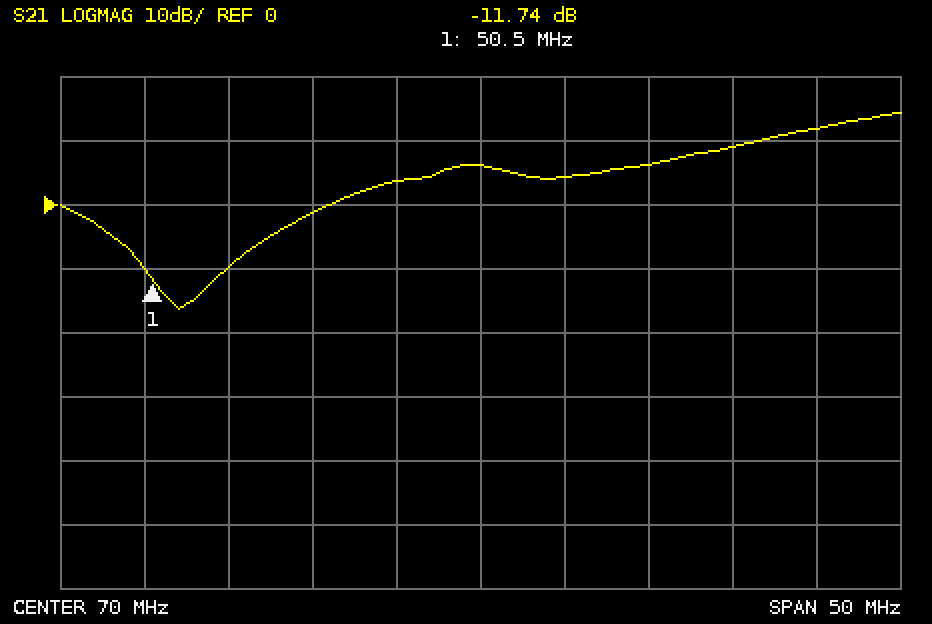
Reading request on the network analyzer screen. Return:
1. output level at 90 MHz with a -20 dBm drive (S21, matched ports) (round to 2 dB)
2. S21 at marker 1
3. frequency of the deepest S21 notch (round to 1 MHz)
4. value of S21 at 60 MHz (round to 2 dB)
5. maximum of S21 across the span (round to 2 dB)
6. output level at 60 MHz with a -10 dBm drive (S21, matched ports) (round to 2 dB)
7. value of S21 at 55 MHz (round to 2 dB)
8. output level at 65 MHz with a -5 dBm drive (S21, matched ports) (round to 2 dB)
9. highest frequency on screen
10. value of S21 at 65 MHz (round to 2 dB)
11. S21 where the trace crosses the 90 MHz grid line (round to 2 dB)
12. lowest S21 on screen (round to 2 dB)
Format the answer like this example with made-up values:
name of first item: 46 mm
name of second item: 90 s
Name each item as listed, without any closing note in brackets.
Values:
output level at 90 MHz with a -20 dBm drive (S21, matched ports): -8 dBm
S21 at marker 1: -11.74 dB
frequency of the deepest S21 notch: 52 MHz
value of S21 at 60 MHz: -2 dB
maximum of S21 across the span: 14 dB
output level at 60 MHz with a -10 dBm drive (S21, matched ports): -12 dBm
value of S21 at 55 MHz: -10 dB
output level at 65 MHz with a -5 dBm drive (S21, matched ports): -2 dBm
highest frequency on screen: 95 MHz
value of S21 at 65 MHz: 4 dB
S21 where the trace crosses the 90 MHz grid line: 12 dB
lowest S21 on screen: -16 dB
